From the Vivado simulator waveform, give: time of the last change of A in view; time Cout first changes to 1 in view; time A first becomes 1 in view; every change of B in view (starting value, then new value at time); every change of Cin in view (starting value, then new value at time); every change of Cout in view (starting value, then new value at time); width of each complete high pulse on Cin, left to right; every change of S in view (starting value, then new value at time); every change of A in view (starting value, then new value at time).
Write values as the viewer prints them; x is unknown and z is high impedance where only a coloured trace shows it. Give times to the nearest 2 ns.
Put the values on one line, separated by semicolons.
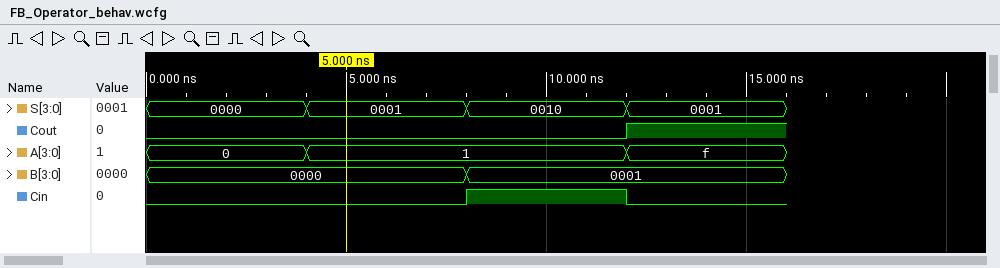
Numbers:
12 ns; 12 ns; 4 ns; 0000, 0001 at 8 ns; 0, 1 at 8 ns, 0 at 12 ns; 0, 1 at 12 ns; 4 ns; 0000, 0001 at 4 ns, 0010 at 8 ns, 0001 at 12 ns; 0, 1 at 4 ns, f at 12 ns
